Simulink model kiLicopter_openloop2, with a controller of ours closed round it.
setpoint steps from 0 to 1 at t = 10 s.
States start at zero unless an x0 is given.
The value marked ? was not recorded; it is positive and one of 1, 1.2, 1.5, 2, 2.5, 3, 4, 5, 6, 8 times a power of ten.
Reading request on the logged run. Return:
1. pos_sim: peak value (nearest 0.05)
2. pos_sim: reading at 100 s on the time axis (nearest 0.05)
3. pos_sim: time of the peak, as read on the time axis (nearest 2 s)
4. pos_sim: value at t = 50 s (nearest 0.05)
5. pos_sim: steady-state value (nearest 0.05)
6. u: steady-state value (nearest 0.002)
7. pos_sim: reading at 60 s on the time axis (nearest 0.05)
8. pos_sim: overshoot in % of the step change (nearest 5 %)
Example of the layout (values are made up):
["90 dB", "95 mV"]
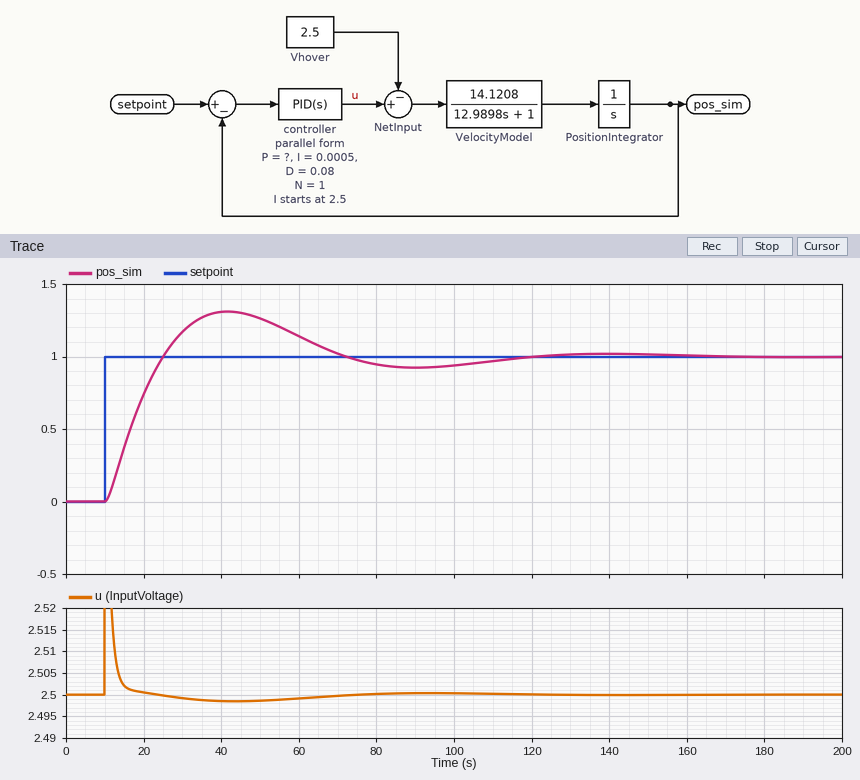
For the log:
["1.30", "0.95", "42 s", "1.25", "1.00", "2.500", "1.15", "30 %"]
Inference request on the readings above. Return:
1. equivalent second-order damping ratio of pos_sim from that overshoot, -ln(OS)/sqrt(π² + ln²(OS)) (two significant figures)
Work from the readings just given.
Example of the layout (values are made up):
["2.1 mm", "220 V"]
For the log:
["0.36"]
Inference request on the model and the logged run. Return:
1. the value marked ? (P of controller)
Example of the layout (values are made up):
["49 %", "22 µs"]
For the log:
["0.01"]
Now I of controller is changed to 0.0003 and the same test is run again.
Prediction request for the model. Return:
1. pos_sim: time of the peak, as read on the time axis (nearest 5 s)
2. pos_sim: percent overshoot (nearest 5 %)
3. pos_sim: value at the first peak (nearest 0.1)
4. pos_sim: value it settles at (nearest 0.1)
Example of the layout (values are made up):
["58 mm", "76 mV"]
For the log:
["45 s", "20 %", "1.2", "1.0"]
